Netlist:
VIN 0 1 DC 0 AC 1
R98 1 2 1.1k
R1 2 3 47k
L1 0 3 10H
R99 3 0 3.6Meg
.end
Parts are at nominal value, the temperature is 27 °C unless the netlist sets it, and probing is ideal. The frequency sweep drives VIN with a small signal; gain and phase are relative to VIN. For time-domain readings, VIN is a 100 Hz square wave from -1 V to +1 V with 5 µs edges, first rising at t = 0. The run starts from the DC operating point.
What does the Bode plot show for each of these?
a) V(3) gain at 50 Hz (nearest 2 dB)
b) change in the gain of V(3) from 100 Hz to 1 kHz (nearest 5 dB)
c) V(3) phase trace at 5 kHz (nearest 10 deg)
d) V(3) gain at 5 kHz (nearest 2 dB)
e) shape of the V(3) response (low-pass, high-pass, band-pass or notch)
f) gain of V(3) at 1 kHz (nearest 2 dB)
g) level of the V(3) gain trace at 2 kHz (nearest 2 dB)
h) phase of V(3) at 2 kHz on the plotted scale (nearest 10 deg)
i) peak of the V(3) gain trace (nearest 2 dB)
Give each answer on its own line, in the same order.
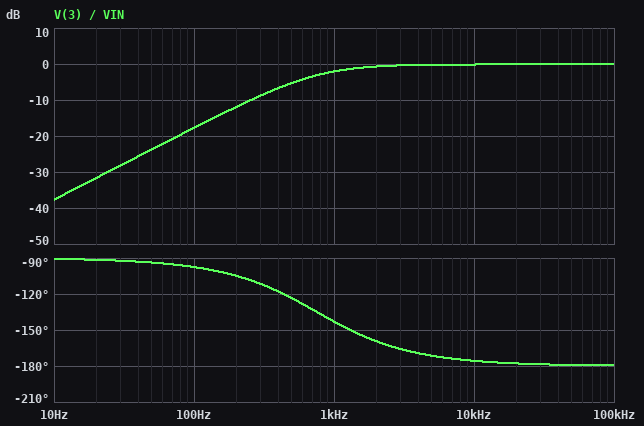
-24 dB
15 dB
-170 deg
0 dB
high-pass
-2 dB
0 dB
-160 deg
0 dB
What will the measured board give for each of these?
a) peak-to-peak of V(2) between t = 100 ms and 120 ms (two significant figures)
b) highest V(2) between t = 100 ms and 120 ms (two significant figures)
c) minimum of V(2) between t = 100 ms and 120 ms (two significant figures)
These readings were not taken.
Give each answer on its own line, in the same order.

2.0 V
1.0 V
-1.0 V
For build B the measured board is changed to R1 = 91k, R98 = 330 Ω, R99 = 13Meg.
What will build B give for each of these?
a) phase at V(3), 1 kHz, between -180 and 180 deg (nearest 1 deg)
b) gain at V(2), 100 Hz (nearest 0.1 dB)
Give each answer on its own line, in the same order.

-125 deg
0 dB
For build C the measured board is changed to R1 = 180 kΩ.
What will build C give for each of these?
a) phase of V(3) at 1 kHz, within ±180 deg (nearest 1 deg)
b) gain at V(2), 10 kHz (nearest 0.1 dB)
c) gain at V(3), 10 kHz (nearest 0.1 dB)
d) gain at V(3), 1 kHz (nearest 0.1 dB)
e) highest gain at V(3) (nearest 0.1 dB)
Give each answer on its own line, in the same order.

-110 deg
0 dB
-0.7 dB
-9.7 dB
-0.4 dB
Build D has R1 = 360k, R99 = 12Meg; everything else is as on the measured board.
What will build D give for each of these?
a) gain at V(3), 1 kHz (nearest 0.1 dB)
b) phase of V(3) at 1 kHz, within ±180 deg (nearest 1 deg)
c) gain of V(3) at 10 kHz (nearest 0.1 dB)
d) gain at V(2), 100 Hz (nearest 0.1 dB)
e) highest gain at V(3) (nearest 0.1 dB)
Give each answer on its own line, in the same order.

-15.3 dB
-100 deg
-1.4 dB
0 dB
-0.3 dB
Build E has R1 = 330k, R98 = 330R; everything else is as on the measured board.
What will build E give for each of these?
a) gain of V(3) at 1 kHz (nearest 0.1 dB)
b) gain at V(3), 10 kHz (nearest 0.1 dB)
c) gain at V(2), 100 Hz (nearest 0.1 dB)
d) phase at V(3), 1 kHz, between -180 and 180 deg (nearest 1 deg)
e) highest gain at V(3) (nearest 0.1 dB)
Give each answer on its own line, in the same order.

-14.6 dB
-1.7 dB
0 dB
-102 deg
-0.8 dB
